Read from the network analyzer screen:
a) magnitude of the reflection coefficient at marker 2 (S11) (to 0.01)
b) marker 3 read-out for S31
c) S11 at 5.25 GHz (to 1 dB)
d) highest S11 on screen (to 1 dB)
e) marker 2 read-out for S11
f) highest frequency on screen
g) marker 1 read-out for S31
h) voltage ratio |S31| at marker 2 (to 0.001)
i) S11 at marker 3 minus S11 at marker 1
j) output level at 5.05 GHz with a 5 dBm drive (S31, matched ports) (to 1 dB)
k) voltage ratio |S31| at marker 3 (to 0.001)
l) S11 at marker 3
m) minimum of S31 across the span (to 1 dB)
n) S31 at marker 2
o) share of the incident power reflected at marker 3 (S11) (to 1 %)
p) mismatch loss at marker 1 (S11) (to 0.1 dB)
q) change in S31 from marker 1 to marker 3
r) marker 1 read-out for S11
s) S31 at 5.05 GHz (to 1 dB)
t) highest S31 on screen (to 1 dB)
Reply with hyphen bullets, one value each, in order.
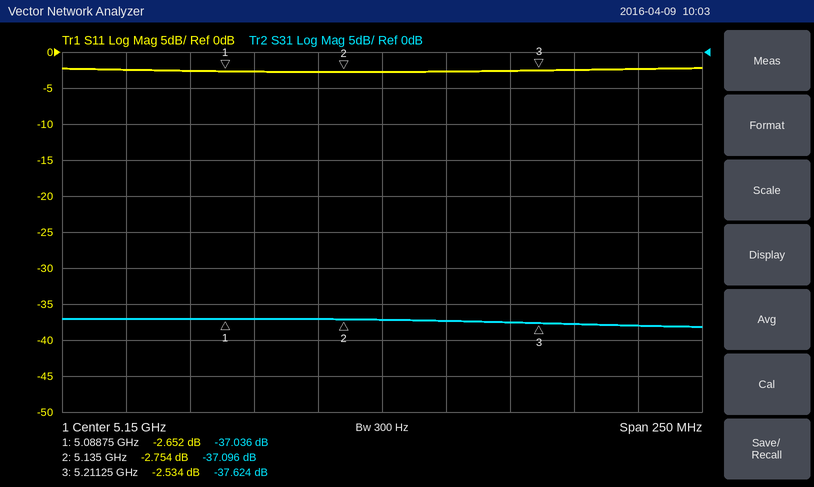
- 0.73
- -37.624 dB
- -2 dB
- -2 dB
- -2.754 dB
- 5.275 GHz
- -37.036 dB
- 0.014
- 0.118 dB
- -32 dBm
- 0.013
- -2.534 dB
- -38 dB
- -37.096 dB
- 56 %
- 3.4 dB
- -0.588 dB
- -2.652 dB
- -37 dB
- -37 dB
